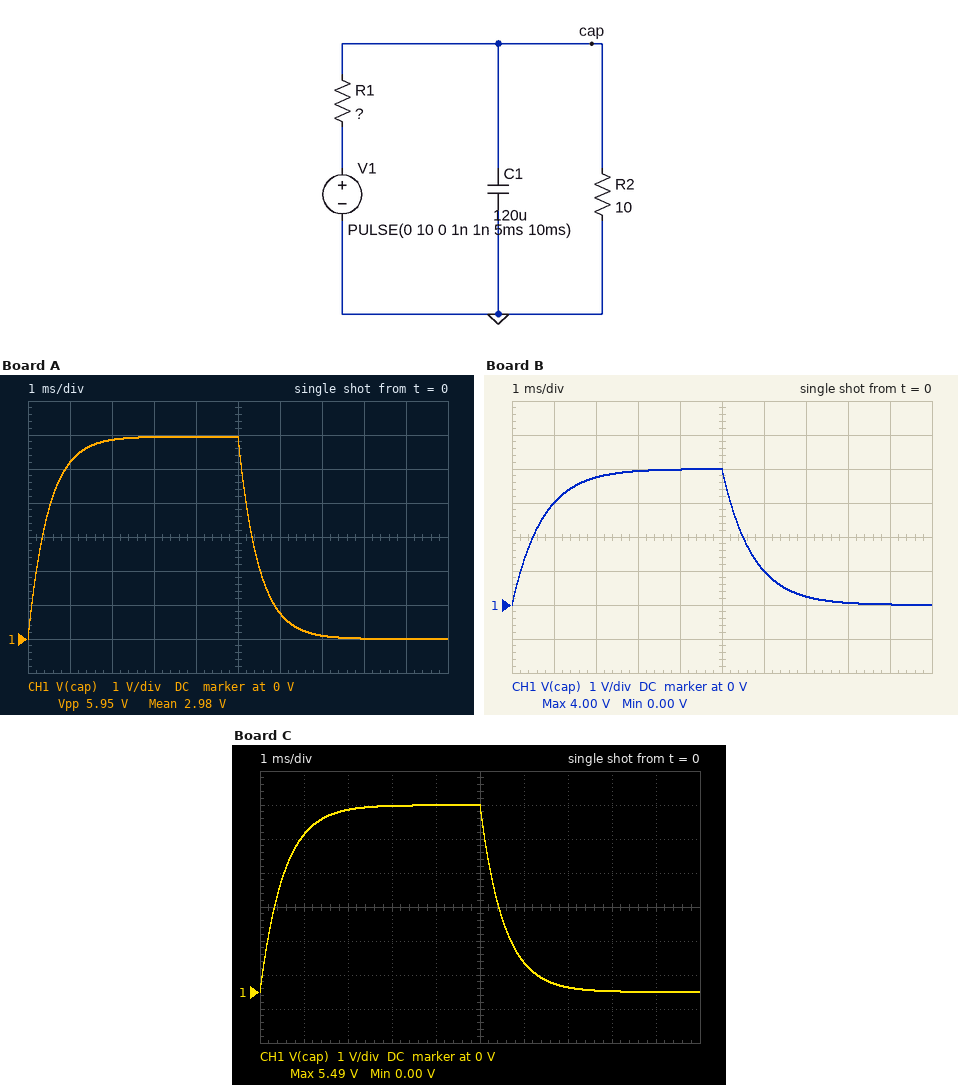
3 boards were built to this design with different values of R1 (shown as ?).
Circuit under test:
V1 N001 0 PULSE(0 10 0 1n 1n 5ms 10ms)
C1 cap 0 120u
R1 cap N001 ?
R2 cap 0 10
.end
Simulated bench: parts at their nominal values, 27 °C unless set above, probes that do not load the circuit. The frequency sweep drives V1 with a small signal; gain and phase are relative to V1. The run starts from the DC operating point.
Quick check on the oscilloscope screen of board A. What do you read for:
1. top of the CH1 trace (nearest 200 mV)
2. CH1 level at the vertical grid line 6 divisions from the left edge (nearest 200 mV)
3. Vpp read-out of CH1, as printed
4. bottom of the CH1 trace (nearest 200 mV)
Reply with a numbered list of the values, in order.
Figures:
1. 6.0 V
2. 800 mV
3. 5.95 V
4. 0 V
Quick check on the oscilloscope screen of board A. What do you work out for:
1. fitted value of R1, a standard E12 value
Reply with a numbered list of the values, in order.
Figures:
1. 6.8 Ω
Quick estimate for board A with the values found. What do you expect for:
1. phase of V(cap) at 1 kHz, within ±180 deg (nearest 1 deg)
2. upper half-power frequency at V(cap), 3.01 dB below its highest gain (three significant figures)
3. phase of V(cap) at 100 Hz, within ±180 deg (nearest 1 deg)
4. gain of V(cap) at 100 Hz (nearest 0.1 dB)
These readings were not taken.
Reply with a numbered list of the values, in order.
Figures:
1. -72 deg
2. 328 Hz
3. -17 deg
4. -4.9 dB
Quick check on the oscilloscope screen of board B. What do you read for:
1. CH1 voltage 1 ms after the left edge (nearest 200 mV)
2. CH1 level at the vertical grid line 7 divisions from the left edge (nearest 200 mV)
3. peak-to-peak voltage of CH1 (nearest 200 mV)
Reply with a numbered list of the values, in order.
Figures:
1. 3.0 V
2. 200 mV
3. 4.0 V
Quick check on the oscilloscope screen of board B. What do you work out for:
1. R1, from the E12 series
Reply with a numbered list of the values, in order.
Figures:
1. 15 Ω
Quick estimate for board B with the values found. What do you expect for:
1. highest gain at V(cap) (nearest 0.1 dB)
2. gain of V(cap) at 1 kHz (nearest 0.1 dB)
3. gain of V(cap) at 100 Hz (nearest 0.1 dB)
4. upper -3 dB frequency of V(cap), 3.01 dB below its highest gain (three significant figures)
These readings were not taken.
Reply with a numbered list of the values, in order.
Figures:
1. -8.0 dB
2. -21.3 dB
3. -8.8 dB
4. 221 Hz
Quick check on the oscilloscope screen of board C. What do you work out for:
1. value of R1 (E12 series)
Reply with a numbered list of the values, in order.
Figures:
1. 8.2 Ω
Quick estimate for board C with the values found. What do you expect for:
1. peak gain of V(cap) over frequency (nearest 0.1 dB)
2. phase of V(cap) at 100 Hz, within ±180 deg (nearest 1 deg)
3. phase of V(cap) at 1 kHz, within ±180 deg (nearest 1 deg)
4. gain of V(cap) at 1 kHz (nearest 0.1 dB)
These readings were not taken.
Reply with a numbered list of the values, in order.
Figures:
1. -5.2 dB
2. -19 deg
3. -74 deg
4. -16.2 dB
